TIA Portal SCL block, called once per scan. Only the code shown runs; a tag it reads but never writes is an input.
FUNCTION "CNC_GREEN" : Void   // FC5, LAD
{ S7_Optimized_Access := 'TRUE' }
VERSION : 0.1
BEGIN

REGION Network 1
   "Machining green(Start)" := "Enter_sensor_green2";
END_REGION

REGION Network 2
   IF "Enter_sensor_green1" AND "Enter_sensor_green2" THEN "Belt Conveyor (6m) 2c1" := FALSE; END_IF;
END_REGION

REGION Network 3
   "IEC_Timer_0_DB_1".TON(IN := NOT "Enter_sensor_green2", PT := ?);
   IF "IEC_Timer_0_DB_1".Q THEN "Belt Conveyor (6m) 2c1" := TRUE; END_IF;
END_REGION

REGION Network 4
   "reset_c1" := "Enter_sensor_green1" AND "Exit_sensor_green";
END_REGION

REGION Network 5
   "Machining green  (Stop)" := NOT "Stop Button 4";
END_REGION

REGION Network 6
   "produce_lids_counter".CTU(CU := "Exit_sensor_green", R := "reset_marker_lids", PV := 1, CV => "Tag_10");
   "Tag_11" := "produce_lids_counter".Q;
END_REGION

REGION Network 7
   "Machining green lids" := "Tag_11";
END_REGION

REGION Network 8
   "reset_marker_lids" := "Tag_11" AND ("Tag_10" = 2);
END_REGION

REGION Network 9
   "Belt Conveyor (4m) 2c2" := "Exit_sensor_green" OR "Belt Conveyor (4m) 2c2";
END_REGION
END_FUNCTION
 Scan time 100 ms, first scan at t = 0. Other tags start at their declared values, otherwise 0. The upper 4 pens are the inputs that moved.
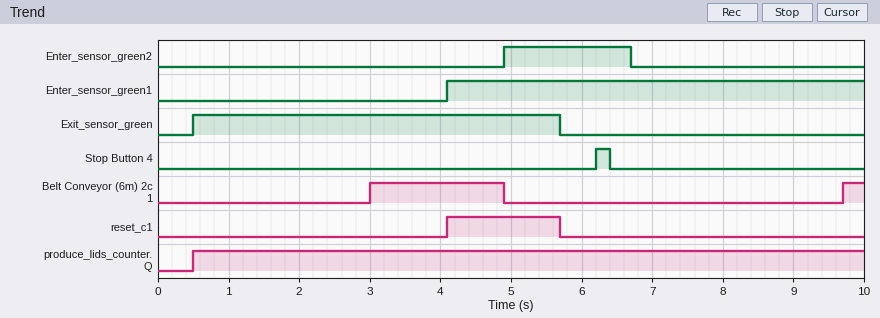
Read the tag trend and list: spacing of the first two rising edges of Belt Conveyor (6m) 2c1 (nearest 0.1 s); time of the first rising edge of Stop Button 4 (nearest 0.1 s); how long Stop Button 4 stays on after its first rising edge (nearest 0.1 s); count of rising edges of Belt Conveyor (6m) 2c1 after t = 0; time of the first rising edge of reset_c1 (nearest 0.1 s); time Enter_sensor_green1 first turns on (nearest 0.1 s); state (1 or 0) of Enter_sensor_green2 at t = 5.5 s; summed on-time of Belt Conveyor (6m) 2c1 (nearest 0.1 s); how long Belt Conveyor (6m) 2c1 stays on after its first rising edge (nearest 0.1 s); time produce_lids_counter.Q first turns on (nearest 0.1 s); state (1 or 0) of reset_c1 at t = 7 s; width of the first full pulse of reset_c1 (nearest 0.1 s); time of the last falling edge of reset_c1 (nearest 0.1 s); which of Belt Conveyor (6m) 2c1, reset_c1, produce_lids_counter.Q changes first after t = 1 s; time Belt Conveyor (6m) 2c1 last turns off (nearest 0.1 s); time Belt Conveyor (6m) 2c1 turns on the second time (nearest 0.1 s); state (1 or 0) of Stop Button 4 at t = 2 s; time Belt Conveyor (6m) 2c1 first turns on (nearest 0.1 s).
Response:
6.7 s
6.2 s
0.2 s
2
4.1 s
4.1 s
1
2.2 s
1.9 s
0.5 s
0
1.6 s
5.7 s
Belt Conveyor (6m) 2c1
4.9 s
9.7 s
0
3.0 s
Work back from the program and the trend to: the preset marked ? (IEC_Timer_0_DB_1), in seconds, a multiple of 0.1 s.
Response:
3.0 s
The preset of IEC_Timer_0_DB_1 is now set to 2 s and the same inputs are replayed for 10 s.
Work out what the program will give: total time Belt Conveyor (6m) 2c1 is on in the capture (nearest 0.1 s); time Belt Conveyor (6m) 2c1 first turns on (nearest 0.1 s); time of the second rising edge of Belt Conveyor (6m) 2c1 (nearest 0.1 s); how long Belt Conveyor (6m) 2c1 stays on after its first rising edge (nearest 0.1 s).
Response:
4.2 s
2.0 s
8.7 s
2.9 s
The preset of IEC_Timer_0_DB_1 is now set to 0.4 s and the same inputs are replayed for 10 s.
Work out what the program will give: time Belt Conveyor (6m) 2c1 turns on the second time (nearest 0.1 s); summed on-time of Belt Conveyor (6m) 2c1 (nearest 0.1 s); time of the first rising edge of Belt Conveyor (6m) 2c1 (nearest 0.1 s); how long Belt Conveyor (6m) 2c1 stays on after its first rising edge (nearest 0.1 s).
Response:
7.1 s
7.4 s
0.4 s
4.5 s
